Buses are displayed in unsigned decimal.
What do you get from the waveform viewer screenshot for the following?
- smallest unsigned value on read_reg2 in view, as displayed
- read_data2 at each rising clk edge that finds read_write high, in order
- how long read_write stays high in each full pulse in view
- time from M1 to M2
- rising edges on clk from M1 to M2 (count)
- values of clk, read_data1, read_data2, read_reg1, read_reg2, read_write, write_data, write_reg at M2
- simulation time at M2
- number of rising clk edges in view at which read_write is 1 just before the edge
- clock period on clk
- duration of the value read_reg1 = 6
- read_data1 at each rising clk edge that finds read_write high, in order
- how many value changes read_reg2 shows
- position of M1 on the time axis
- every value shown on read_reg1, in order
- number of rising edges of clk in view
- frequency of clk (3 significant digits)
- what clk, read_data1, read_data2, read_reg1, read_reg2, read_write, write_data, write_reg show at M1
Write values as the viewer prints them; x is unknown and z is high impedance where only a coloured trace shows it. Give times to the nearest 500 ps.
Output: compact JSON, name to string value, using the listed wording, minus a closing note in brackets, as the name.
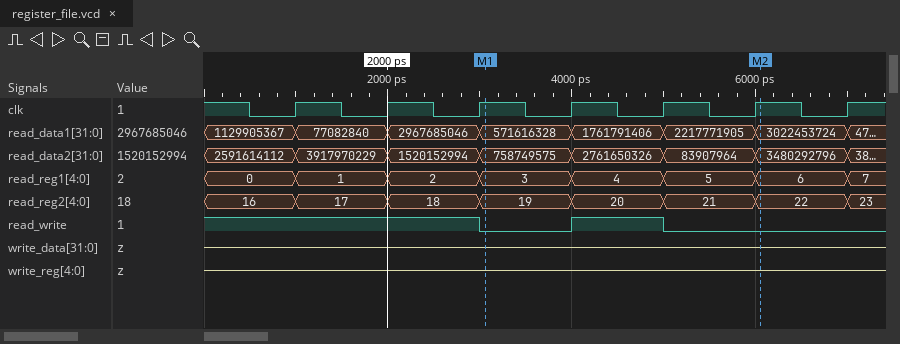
{"smallest unsigned value on read_reg2 in view, as displayed": "16", "read_data2 at each rising clk edge that finds read_write high, in order": "2591614112, 3917970229, 1520152994, 2761650326", "how long read_write stays high in each full pulse in view": "1000 ps", "time from M1 to M2": "3000 ps", "rising edges on clk from M1 to M2": "3", "values of clk, read_data1, read_data2, read_reg1, read_reg2, read_write, write_data, write_reg at M2": "clk=1, read_data1=3022453724, read_data2=3480292796, read_reg1=6, read_reg2=22, read_write=0, write_data=z, write_reg=z", "simulation time at M2": "6000 ps", "number of rising clk edges in view at which read_write is 1 just before the edge": "4", "clock period on clk": "1000 ps", "duration of the value read_reg1 = 6": "1000 ps", "read_data1 at each rising clk edge that finds read_write high, in order": "1129905367, 77082840, 2967685046, 1761791406", "how many value changes read_reg2 shows": "7", "position of M1 on the time axis": "3000 ps", "every value shown on read_reg1, in order": "0, 1, 2, 3, 4, 5, 6, 7", "number of rising edges of clk in view": "7", "frequency of clk": "1.00 GHz", "what clk, read_data1, read_data2, read_reg1, read_reg2, read_write, write_data, write_reg show at M1": "clk=1, read_data1=571616328, read_data2=758749575, read_reg1=3, read_reg2=19, read_write=0, write_data=z, write_reg=z"}
